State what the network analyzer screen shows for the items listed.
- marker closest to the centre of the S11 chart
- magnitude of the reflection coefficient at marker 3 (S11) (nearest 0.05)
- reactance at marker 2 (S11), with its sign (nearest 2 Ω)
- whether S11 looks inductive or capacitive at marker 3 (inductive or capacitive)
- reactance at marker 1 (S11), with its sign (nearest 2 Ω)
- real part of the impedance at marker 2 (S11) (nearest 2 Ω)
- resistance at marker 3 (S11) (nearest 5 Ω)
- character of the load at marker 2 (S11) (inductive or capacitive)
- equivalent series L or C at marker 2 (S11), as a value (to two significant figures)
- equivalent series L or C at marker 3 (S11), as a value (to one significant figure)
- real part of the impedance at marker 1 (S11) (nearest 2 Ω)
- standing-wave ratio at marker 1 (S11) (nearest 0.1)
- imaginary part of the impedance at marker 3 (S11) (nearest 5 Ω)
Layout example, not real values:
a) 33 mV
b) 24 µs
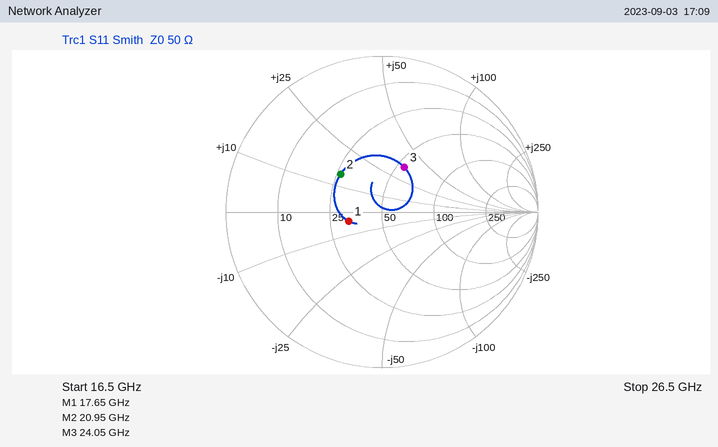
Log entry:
a) marker 1
b) 0.30
c) +14 Ω
d) inductive
e) -4 Ω
f) 26 Ω
g) 55 Ω
h) inductive
i) 110 pH
j) 200 pH
k) 32 Ω
l) 1.6
m) +35 Ω
